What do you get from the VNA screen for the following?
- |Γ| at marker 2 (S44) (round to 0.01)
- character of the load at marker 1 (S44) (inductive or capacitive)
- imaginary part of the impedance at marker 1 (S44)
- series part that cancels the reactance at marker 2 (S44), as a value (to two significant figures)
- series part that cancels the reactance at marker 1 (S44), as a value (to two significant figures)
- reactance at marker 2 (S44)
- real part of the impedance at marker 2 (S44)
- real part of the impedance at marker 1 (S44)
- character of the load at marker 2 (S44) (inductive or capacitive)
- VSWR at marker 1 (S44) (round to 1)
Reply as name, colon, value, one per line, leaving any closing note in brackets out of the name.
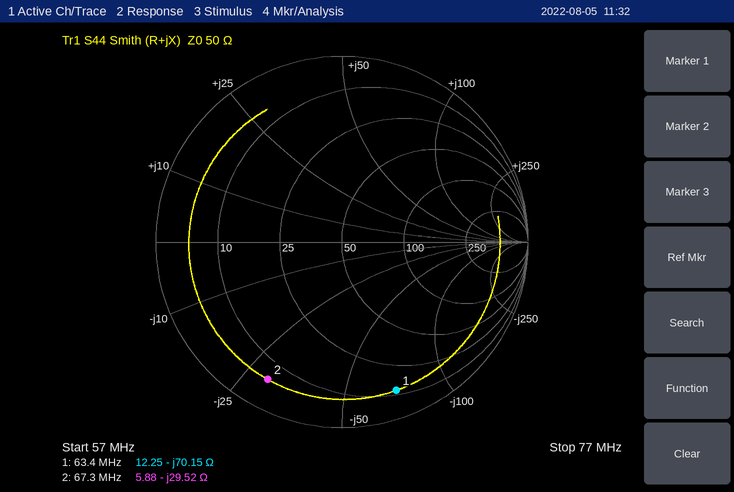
|Γ| at marker 2 (S44): 0.84
character of the load at marker 1 (S44): capacitive
imaginary part of the impedance at marker 1: -70.15 Ω
series part that cancels the reactance at marker 2 (S44), as a value: 70 nH
series part that cancels the reactance at marker 1 (S44), as a value: 180 nH
reactance at marker 2: -29.52 Ω
real part of the impedance at marker 2: 5.88 Ω
real part of the impedance at marker 1: 12.25 Ω
character of the load at marker 2 (S44): capacitive
VSWR at marker 1 (S44): 12
